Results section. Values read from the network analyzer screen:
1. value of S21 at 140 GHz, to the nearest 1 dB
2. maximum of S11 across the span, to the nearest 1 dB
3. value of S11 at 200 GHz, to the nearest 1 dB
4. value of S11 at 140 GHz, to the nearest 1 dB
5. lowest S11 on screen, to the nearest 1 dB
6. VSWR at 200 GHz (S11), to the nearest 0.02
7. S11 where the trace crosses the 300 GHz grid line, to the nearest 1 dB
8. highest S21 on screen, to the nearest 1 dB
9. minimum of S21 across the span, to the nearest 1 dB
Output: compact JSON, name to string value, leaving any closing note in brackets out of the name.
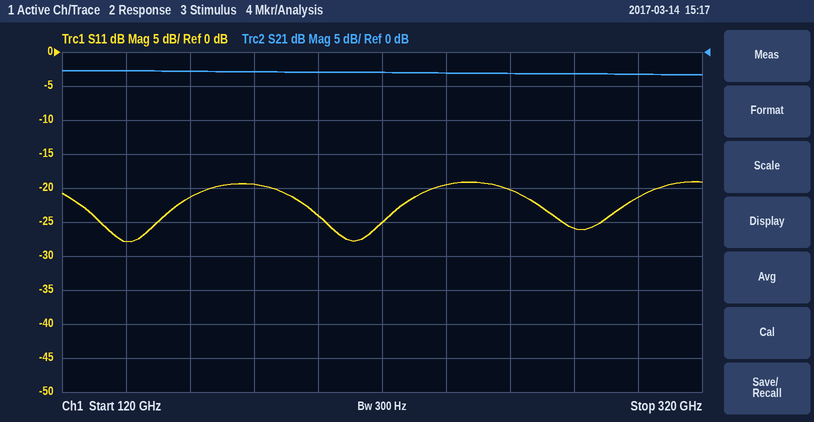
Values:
{"value of S21 at 140 GHz, to the nearest 1 dB": "-3 dB", "maximum of S11 across the span, to the nearest 1 dB": "-19 dB", "value of S11 at 200 GHz, to the nearest 1 dB": "-24 dB", "value of S11 at 140 GHz, to the nearest 1 dB": "-28 dB", "lowest S11 on screen, to the nearest 1 dB": "-28 dB", "VSWR at 200 GHz (S11), to the nearest 0.02": "1.14", "S11 where the trace crosses the 300 GHz grid line, to the nearest 1 dB": "-21 dB", "highest S21 on screen, to the nearest 1 dB": "-3 dB", "minimum of S21 across the span, to the nearest 1 dB": "-3 dB"}
